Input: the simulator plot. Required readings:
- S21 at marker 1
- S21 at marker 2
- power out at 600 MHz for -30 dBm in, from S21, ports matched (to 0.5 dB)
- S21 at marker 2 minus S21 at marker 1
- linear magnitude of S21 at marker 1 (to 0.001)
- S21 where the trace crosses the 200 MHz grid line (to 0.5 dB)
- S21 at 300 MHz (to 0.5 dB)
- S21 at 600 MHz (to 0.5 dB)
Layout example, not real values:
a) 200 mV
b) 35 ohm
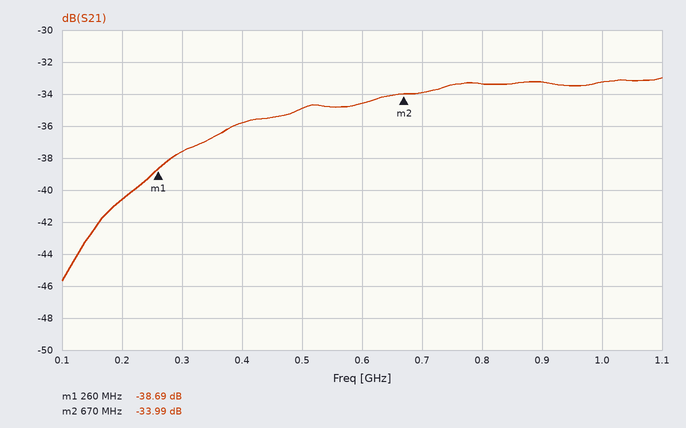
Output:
a) -38.69 dB
b) -33.99 dB
c) -64.5 dBm
d) 4.70 dB
e) 0.012
f) -40.5 dB
g) -37.5 dB
h) -34.5 dB
